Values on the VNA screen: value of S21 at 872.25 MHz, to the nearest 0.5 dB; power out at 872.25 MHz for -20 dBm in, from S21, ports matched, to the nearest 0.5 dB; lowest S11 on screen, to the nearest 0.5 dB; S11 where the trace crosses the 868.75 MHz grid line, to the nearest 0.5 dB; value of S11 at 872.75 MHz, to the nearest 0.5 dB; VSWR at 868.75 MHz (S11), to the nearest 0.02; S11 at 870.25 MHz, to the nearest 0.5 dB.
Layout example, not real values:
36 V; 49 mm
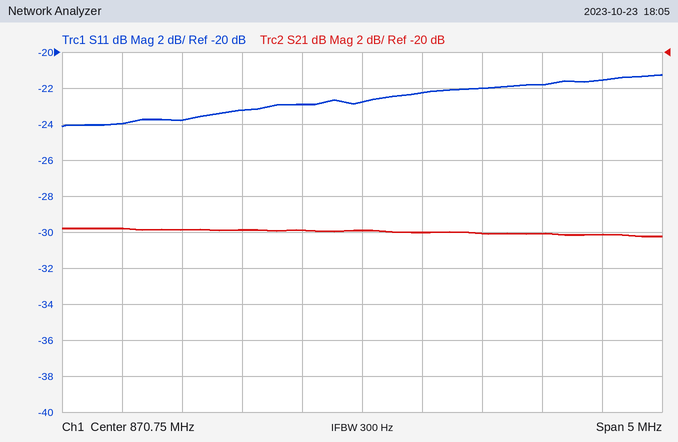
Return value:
-30.0 dB; -50.0 dBm; -24.0 dB; -24.0 dB; -21.5 dB; 1.14; -23.0 dB
